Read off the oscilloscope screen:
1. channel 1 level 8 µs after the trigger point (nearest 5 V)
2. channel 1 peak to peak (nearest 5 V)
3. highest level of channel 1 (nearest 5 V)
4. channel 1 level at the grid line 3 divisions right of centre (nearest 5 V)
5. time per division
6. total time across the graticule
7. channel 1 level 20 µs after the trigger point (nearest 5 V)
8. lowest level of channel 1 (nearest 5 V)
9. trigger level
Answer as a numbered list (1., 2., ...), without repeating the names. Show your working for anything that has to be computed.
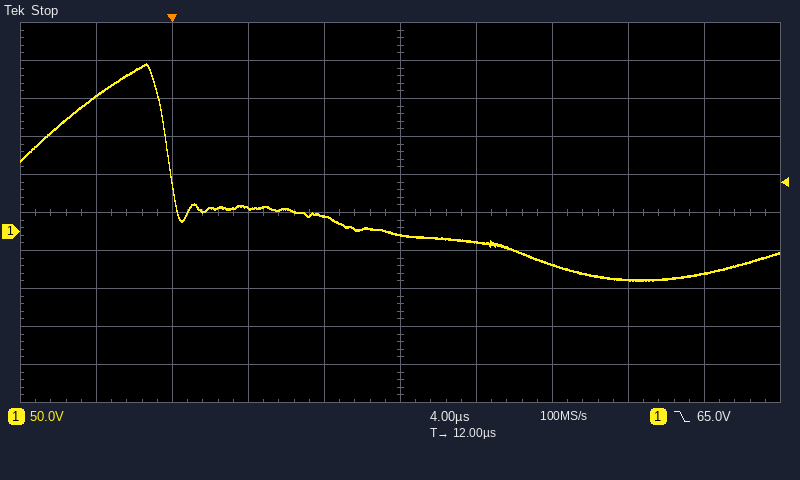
1. 20 V
2. 220 V − (-65 V) = 285 V
3. 220 V
4. -65 V
5. 4 µs
6. 40 µs
7. -45 V
8. -65 V
9. 65.0 V
